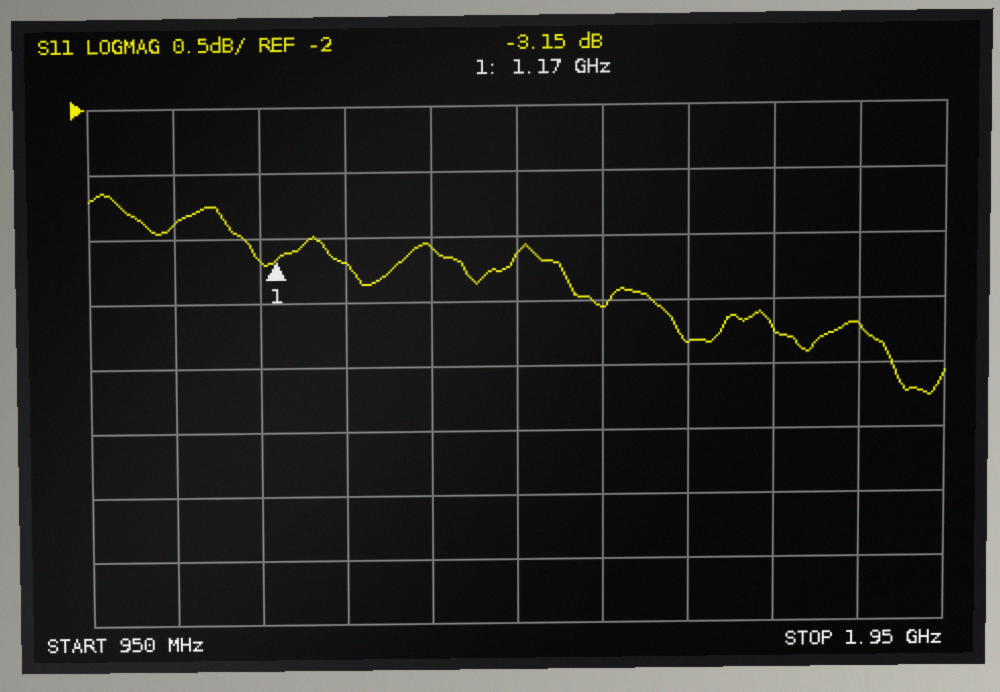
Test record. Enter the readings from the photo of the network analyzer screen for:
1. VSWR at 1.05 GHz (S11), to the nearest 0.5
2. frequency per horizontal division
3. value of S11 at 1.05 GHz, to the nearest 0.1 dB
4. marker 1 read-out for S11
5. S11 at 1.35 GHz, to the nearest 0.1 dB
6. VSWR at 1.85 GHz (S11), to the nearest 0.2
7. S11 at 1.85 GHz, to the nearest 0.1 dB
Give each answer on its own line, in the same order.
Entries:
6.0
100 MHz
-2.9 dB
-3.15 dB
-3.1 dB
4.8
-3.7 dB
